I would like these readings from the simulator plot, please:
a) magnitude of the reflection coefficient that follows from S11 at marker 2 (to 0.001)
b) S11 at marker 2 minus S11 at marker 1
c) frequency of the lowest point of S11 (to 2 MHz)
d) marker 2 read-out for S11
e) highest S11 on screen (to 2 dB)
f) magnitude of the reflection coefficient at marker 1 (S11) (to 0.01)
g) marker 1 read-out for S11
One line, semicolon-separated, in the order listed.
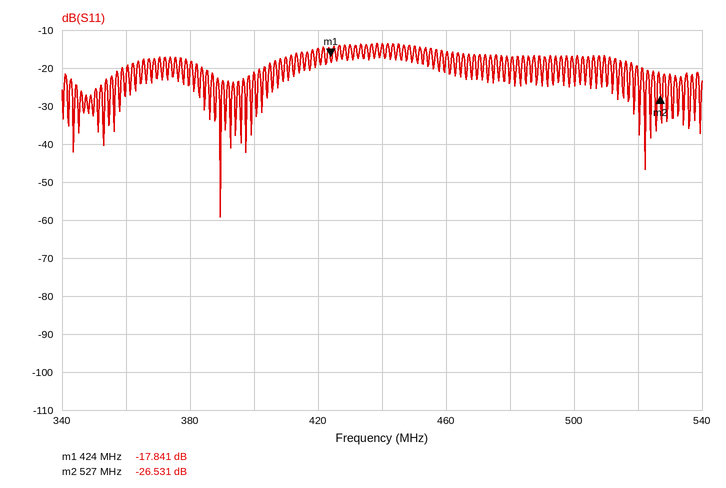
0.047; -8.690 dB; 390 MHz; -26.531 dB; -14 dB; 0.13; -17.841 dB
